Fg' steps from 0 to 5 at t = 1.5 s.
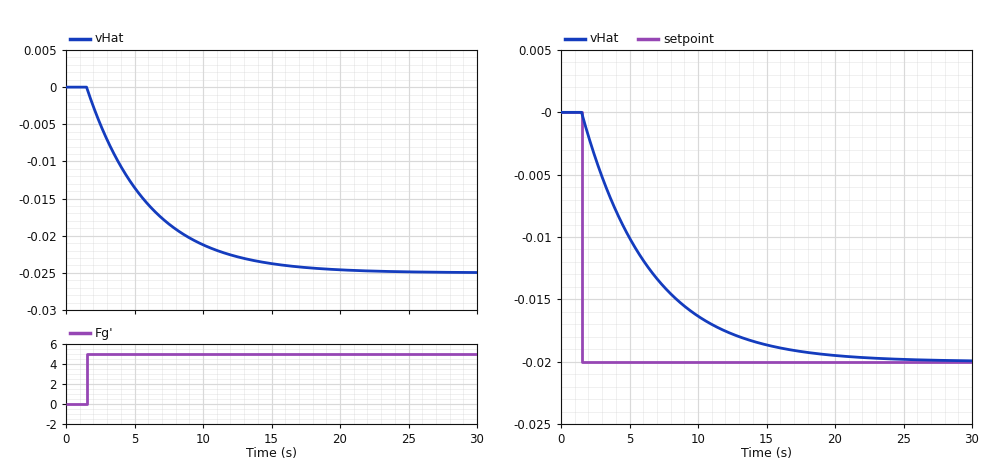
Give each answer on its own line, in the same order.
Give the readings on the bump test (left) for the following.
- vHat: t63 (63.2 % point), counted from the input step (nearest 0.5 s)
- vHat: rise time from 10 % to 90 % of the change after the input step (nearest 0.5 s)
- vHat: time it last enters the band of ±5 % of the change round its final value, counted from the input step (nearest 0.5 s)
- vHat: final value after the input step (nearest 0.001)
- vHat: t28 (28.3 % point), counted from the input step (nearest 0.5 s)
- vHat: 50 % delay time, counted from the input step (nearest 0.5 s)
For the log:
4.5 s
10.0 s
13.5 s
-0.025
1.5 s
3.0 s
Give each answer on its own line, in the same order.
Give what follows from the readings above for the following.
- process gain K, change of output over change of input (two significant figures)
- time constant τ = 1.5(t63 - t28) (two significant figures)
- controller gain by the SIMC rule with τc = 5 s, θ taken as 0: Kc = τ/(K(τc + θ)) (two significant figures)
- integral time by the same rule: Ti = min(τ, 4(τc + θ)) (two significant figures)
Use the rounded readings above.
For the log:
-0.0050
4.5 s
-180
4.5 s
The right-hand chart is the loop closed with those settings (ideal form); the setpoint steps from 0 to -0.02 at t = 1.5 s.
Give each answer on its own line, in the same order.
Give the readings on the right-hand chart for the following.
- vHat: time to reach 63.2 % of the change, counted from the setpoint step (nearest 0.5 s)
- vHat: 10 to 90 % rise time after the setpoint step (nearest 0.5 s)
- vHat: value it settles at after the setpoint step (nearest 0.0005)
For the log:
5.0 s
11.0 s
-0.0200
